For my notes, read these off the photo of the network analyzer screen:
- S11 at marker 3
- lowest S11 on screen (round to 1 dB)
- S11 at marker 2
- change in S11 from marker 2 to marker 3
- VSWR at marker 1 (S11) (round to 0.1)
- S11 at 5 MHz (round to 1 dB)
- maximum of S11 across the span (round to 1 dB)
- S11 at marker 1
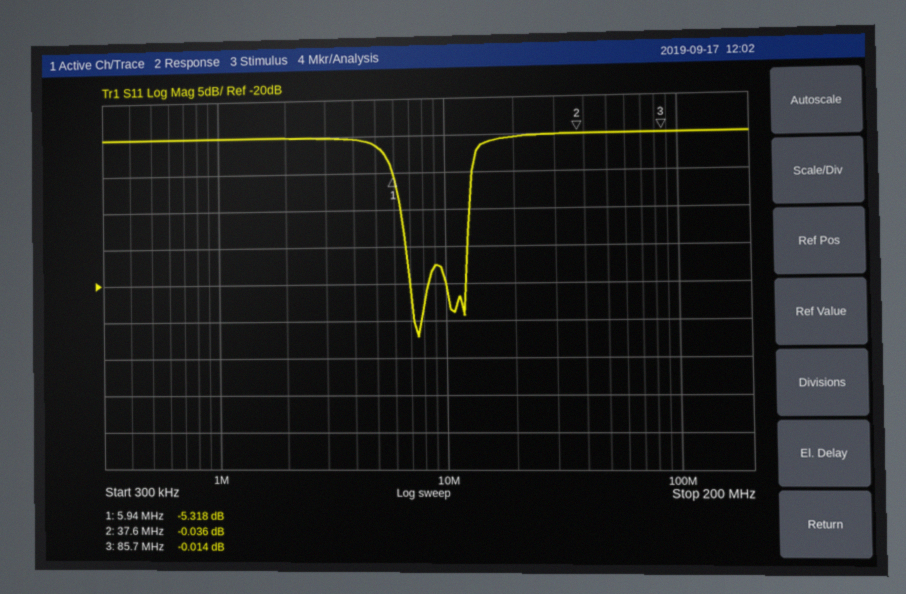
-0.014 dB
-27 dB
-0.036 dB
0.022 dB
3.4
-1 dB
0 dB
-5.318 dB
